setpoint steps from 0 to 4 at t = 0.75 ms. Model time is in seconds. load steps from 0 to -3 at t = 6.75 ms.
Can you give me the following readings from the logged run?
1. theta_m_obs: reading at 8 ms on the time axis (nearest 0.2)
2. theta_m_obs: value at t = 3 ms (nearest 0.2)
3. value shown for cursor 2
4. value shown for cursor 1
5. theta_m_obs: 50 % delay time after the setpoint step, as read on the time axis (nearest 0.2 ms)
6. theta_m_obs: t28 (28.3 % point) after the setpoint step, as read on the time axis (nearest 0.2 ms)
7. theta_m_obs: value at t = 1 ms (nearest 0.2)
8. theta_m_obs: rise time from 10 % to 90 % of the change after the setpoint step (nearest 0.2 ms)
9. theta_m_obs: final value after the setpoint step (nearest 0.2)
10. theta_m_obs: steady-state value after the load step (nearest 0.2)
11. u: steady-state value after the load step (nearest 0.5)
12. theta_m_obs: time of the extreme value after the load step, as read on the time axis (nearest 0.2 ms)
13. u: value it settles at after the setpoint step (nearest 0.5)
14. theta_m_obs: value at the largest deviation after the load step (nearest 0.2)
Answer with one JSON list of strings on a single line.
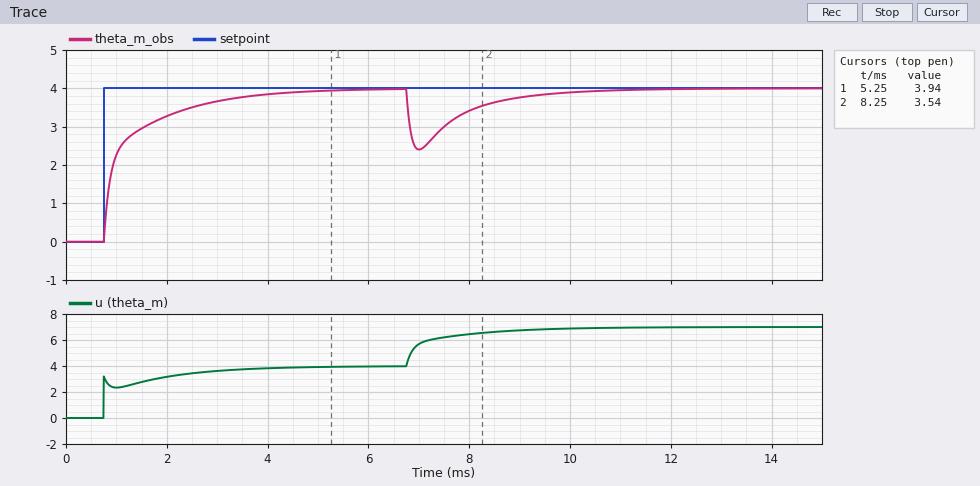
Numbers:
["3.4", "3.6", "3.54", "3.94", "1.0 ms", "0.8 ms", "2.2", "2.0 ms", "4.0", "4.0", "7.0", "7.0 ms", "4.0", "2.4"]
